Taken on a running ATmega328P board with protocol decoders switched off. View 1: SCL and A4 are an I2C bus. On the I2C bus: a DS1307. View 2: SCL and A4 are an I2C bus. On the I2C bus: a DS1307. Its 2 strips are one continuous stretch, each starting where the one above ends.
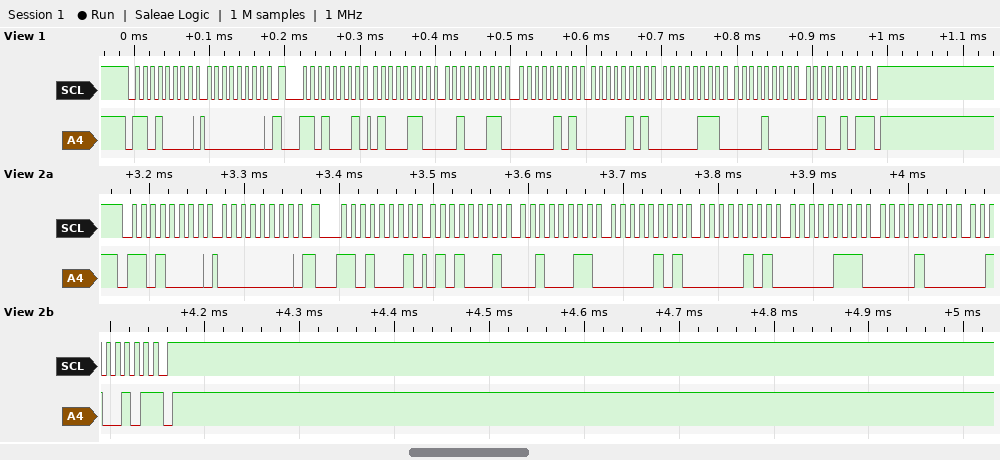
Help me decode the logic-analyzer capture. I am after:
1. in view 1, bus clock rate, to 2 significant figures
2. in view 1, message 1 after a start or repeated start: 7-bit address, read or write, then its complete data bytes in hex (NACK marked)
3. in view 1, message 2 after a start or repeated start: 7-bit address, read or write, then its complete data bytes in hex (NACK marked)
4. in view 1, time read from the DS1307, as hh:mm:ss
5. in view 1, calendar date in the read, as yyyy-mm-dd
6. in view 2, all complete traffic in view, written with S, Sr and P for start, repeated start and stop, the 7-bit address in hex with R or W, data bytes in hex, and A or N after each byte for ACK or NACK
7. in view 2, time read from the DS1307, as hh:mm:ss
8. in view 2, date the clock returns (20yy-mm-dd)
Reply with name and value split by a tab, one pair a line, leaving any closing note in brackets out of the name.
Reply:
in view 1, bus clock rate, to 2 significant figures	100 kHz
in view 1, message 1 after a start or repeated start: 7-bit address, read or write, then its complete data bytes in hex	0x68 write: 00
in view 1, message 2 after a start or repeated start: 7-bit address, read or write, then its complete data bytes in hex	0x68 read: 46 23 05 05 07 08 25 NACK
in view 1, time read from the DS1307, as hh:mm:ss	05:23:46
in view 1, calendar date in the read, as yyyy-mm-dd	2025-08-07
in view 2, all complete traffic in view, written with S, Sr and P for start, repeated start and stop, the 7-bit address in hex with R or W, data bytes in hex, and A or N after each byte for ACK or NACK	S 68W A 00 A Sr 68R A 51 A 23 A 05 A 05 A 07 A 08 A 25 N P
in view 2, time read from the DS1307, as hh:mm:ss	05:23:51
in view 2, date the clock returns	2025-08-07
